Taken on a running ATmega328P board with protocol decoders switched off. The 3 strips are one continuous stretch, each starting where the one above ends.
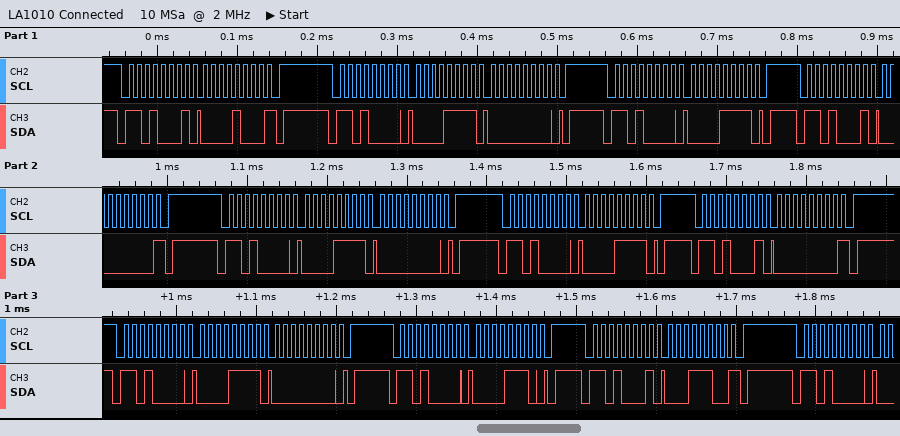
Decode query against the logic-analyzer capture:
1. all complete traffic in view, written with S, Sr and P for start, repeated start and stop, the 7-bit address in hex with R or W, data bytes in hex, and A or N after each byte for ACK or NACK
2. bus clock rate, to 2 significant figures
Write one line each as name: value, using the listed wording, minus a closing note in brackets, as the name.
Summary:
all complete traffic in view, written with S, Sr and P for start, repeated start and stop, the 7-bit address in hex with R or W, data bytes in hex, and A or N after each byte for ACK or NACK: S 68R A 08 N P S 68W A 0F A 00 A P S 68W A 0F A P S 68R A 00 N P S 68W A 0F A 00 A P S 68W A 0F A P S 68R A 00 N P S 68W A 0F A 00 A P S 68W A 0E A P S 68R A 1C N P S 68W A
bus clock rate, to 2 significant figures: 100 kHz
